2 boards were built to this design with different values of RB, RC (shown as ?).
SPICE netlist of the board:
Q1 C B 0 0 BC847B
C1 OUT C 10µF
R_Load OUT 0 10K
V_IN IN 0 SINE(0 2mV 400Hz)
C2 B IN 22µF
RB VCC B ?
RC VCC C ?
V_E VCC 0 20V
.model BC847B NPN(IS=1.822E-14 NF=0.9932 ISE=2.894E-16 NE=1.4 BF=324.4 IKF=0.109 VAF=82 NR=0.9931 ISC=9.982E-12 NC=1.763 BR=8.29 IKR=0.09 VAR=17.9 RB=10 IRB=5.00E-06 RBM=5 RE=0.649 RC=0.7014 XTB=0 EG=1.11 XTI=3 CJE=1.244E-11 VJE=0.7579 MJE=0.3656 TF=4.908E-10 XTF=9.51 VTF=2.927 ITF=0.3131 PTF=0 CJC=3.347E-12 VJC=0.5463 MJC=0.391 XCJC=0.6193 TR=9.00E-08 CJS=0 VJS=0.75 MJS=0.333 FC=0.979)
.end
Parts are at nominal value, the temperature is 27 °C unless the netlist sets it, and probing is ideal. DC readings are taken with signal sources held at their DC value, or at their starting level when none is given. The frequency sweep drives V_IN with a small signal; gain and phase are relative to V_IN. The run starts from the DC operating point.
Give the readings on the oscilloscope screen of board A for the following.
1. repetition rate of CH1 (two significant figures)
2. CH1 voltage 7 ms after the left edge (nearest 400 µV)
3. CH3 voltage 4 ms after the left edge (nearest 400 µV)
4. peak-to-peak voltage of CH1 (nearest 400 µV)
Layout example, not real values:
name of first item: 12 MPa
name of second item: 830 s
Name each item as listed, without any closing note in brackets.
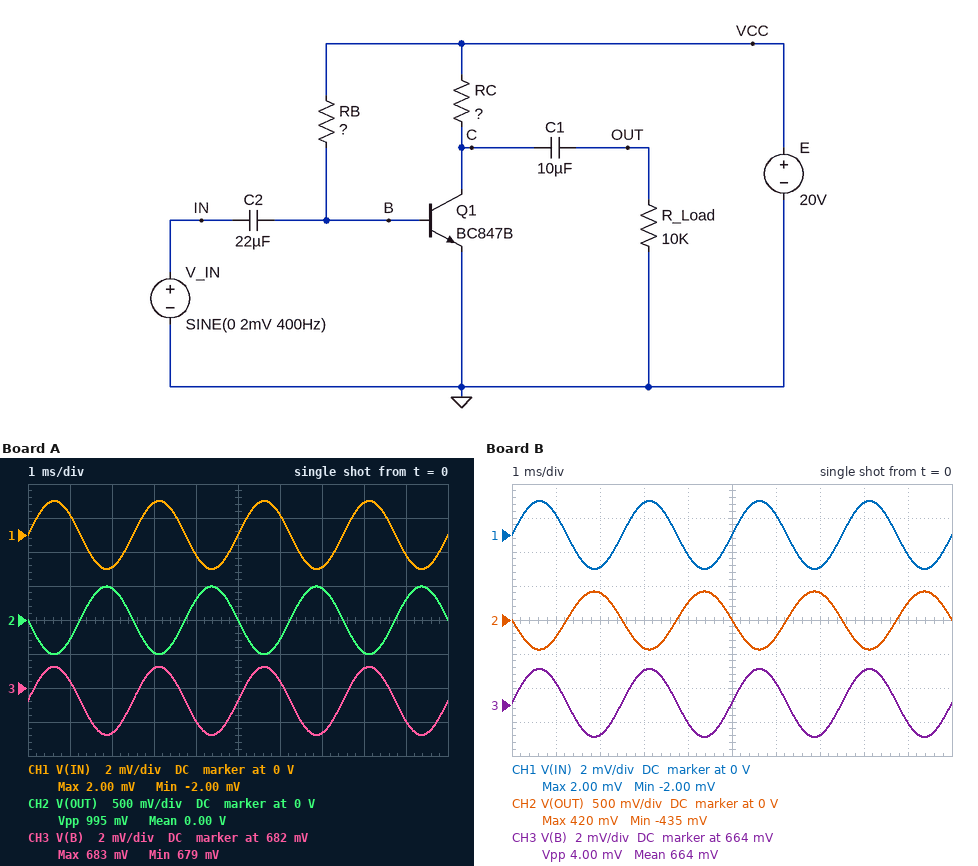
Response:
repetition rate of CH1: 400 Hz
CH1 voltage 7 ms after the left edge: -2.0 mV
CH3 voltage 4 ms after the left edge: 680.0 mV
peak-to-peak voltage of CH1: 4.0 mV
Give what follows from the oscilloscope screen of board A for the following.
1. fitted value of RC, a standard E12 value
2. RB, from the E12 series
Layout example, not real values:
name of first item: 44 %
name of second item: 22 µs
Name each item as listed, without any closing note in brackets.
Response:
fitted value of RC, a standard E12 value: 1.8 kΩ
RB, from the E12 series: 1.2 MΩ
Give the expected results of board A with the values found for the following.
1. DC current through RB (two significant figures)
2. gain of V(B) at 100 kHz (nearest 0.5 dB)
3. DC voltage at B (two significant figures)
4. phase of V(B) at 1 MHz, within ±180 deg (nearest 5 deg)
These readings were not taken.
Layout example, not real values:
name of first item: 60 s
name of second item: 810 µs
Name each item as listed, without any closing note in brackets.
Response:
DC current through RB: 16 µA
gain of V(B) at 100 kHz: 0 dB
DC voltage at B: 680 mV
phase of V(B) at 1 MHz, within ±180 deg: 0 deg
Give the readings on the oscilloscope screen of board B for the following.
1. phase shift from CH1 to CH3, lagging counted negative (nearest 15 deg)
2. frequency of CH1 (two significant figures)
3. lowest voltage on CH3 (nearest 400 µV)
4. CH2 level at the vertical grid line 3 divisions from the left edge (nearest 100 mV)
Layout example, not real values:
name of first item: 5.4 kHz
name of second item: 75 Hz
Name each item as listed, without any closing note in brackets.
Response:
phase shift from CH1 to CH3, lagging counted negative: 0 deg
frequency of CH1: 400 Hz
lowest voltage on CH3: 662.0 mV
CH2 level at the vertical grid line 3 divisions from the left edge: -400 mV
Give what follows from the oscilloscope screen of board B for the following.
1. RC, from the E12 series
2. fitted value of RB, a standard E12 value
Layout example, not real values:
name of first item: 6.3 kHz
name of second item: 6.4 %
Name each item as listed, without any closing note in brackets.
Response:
RC, from the E12 series: 2.7 kΩ
fitted value of RB, a standard E12 value: 2.2 MΩ
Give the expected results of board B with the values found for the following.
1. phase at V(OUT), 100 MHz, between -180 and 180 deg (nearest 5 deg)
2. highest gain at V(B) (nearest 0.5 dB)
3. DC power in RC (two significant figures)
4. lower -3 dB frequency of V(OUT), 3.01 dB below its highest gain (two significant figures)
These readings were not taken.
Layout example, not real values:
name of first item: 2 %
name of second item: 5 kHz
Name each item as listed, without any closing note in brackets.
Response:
phase at V(OUT), 100 MHz, between -180 and 180 deg: 105 deg
highest gain at V(B): 0 dB
DC power in RC: 25 mW
lower -3 dB frequency of V(OUT), 3.01 dB below its highest gain: 2.8 Hz
